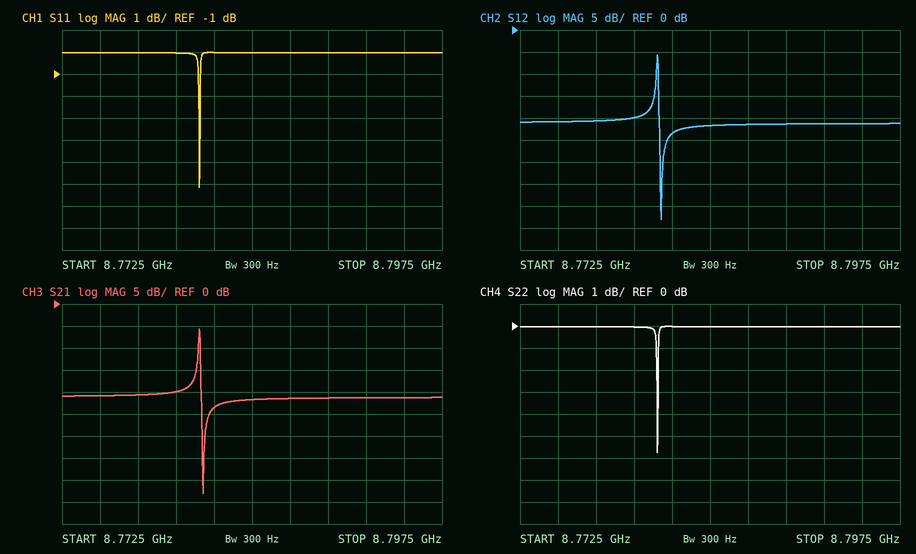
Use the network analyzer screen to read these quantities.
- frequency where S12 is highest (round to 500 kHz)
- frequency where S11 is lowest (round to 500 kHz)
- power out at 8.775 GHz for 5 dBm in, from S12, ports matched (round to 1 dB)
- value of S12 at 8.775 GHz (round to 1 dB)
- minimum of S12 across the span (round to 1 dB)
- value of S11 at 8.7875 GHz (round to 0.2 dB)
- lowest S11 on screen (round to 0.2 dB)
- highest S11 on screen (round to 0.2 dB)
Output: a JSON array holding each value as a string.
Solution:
["8.7815 GHz", "8.7815 GHz", "-16 dBm", "-21 dB", "-43 dB", "0.0 dB", "-6.2 dB", "0.0 dB"]
